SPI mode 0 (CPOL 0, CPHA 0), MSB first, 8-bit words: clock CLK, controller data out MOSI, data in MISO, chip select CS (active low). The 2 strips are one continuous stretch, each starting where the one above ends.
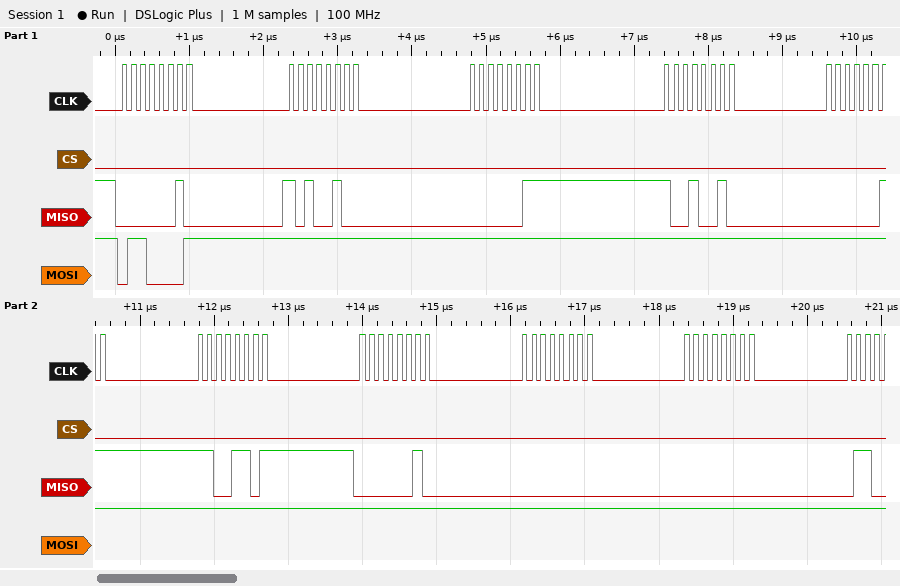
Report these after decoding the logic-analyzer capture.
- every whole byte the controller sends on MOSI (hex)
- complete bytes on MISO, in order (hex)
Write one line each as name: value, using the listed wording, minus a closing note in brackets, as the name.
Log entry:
every whole byte the controller sends on MOSI: 61 FF FF FF FF FF FF FF FF
complete bytes on MISO, in order: 02 A4 03 92 03 CD 02 00 00
